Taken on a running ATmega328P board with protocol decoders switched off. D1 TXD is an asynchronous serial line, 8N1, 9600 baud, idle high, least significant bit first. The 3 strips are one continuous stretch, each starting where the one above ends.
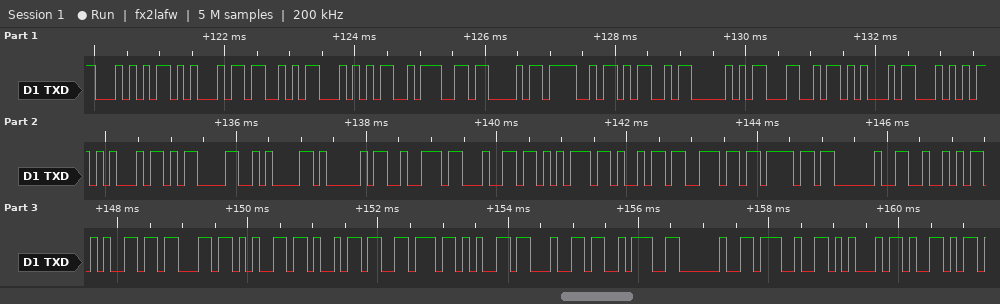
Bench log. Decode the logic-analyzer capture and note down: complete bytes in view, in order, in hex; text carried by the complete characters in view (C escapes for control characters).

54 45 53 54 3A 43 4F 4D 50 4C 45 54 45 0D 0A 41 72 64 75 69 6E 6F 20 52 65 63 65 69 76 65 64 3A 20 27 45 59
"TEST:COMPLETE\r\nArduino Received: 'EY"
